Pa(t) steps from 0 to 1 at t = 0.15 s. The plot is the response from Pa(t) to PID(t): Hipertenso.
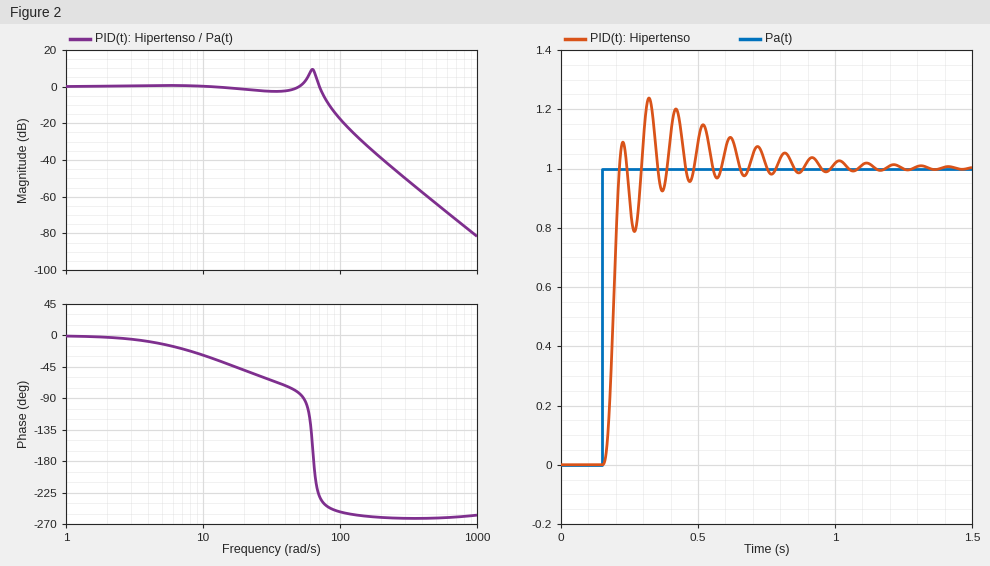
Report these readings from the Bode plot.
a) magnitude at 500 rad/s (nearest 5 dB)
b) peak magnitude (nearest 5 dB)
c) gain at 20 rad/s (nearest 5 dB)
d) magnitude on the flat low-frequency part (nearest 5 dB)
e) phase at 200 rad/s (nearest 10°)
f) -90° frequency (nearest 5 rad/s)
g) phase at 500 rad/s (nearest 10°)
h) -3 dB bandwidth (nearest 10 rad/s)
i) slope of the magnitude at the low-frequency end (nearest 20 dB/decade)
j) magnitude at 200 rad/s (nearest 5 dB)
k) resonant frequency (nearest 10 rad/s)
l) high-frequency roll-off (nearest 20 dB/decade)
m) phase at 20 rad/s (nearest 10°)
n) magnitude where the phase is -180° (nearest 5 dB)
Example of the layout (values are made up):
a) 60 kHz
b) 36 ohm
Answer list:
a) -65 dB
b) 10 dB
c) 0 dB
d) 0 dB
e) -260°
f) 55 rad/s
g) -260°
h) 70 rad/s
i) 0 dB/decade
j) -40 dB
k) 60 rad/s
l) -60 dB/decade
m) -50°
n) 10 dB
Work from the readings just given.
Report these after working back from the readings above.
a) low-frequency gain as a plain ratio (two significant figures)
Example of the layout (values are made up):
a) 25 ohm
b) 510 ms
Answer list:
a) 1.0
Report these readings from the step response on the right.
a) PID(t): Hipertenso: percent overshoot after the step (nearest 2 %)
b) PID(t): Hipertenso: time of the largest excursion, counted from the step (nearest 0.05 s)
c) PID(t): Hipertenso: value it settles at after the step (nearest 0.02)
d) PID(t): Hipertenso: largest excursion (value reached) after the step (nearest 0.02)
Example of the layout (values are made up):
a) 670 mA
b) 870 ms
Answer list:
a) 24 %
b) 0.15 s
c) 1.00
d) 1.24
